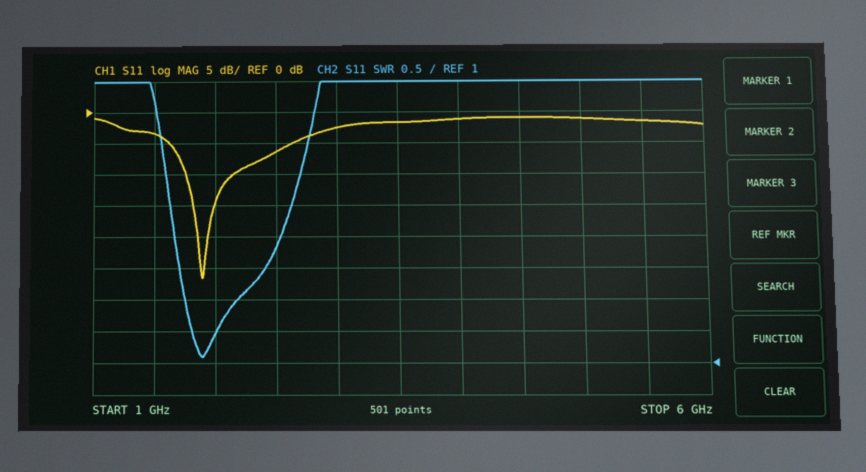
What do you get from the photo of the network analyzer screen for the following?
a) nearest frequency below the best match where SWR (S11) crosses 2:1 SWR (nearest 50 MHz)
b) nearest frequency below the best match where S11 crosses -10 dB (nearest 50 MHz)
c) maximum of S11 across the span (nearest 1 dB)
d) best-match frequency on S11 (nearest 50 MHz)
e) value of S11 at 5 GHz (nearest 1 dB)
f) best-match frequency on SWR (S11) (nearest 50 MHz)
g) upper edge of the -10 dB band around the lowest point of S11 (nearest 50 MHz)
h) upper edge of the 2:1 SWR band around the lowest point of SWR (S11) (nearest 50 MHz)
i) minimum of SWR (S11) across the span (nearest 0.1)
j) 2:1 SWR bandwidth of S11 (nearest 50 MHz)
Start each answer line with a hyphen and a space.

- 1.75 GHz
- 1.75 GHz
- -1 dB
- 1.90 GHz
- -1 dB
- 1.90 GHz
- 2.15 GHz
- 2.20 GHz
- 1.1
- 450 MHz
